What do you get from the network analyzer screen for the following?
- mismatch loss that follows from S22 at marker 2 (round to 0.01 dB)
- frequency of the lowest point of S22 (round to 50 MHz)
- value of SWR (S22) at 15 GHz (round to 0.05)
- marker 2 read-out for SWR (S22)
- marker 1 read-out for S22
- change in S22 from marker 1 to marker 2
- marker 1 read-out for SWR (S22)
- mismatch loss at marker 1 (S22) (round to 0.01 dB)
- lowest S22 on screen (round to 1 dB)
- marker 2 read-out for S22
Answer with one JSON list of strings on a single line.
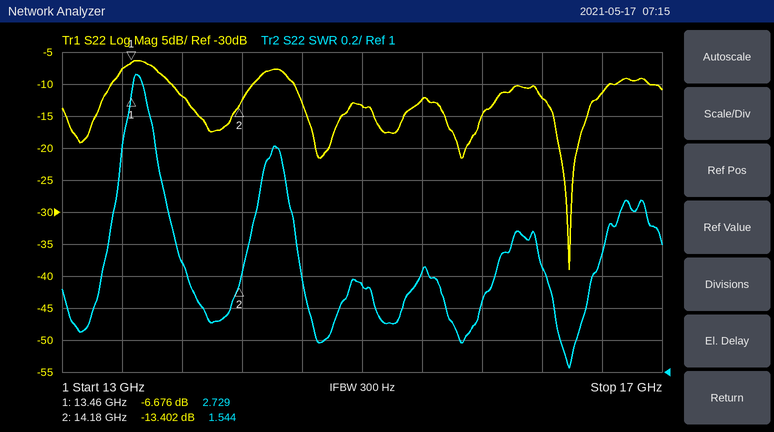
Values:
["0.20 dB", "16.40 GHz", "1.55", "1.544", "-6.676 dB", "-6.726 dB", "2.729", "1.05 dB", "-39 dB", "-13.402 dB"]
